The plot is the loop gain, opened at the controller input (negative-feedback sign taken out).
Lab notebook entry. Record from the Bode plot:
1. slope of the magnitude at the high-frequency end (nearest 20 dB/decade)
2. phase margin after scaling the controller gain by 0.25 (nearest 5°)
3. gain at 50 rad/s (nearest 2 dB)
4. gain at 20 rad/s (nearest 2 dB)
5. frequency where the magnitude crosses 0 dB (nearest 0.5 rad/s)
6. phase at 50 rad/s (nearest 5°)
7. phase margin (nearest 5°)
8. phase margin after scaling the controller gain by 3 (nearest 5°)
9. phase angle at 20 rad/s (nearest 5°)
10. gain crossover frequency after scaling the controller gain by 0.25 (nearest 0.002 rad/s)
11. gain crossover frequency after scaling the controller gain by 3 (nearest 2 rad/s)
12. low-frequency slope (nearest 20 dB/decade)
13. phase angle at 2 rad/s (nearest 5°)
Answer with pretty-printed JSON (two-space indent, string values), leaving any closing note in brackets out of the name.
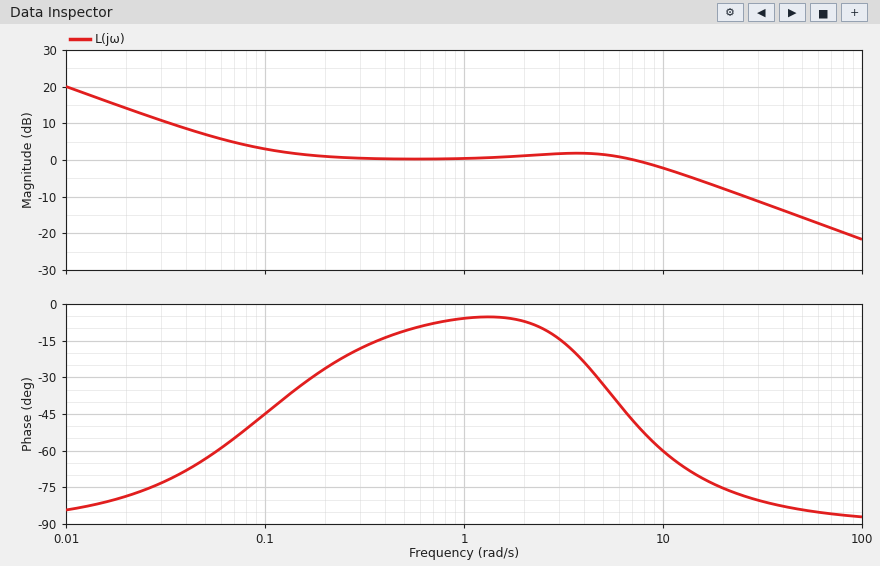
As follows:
{
  "slope of the magnitude at the high-frequency end": "-20 dB/decade",
  "phase margin after scaling the controller gain by 0.25": "105°",
  "gain at 50 rad/s": "-16 dB",
  "gain at 20 rad/s": "-8 dB",
  "frequency where the magnitude crosses 0 dB": "7.0 rad/s",
  "phase at 50 rad/s": "-85°",
  "phase margin": "130°",
  "phase margin after scaling the controller gain by 3": "100°",
  "phase angle at 20 rad/s": "-75°",
  "gain crossover frequency after scaling the controller gain by 0.25": "0.026 rad/s",
  "gain crossover frequency after scaling the controller gain by 3": "24 rad/s",
  "low-frequency slope": "-20 dB/decade",
  "phase angle at 2 rad/s": "-5°"
}
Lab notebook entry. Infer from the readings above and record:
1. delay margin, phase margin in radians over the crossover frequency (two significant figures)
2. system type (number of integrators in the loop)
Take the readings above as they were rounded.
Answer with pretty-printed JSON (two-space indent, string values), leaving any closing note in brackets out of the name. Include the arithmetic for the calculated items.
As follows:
{
  "delay margin, phase margin in radians over the crossover frequency": "130 × π / 180 / 7 = 0.32 s",
  "system type": "1"
}
